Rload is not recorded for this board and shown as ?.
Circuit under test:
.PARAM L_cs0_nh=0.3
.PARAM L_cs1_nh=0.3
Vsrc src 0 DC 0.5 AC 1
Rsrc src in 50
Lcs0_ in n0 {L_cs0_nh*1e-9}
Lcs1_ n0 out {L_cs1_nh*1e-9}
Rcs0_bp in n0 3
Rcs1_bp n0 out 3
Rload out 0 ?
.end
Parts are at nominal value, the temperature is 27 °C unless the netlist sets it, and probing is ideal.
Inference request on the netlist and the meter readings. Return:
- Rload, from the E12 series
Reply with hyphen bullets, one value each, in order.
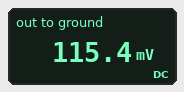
- 15 Ω
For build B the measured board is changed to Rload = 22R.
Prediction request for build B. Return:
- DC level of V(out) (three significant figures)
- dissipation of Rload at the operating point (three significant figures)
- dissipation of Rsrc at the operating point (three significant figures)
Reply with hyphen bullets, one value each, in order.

- 153 mV
- 1.06 mW
- 2.41 mW
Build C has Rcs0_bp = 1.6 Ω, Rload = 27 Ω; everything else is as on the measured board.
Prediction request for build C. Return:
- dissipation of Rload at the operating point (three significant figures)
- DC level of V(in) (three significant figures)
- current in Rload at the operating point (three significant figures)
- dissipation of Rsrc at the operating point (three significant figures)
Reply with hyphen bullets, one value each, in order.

- 1.14 mW
- 175 mV
- 6.49 mA
- 2.11 mW
